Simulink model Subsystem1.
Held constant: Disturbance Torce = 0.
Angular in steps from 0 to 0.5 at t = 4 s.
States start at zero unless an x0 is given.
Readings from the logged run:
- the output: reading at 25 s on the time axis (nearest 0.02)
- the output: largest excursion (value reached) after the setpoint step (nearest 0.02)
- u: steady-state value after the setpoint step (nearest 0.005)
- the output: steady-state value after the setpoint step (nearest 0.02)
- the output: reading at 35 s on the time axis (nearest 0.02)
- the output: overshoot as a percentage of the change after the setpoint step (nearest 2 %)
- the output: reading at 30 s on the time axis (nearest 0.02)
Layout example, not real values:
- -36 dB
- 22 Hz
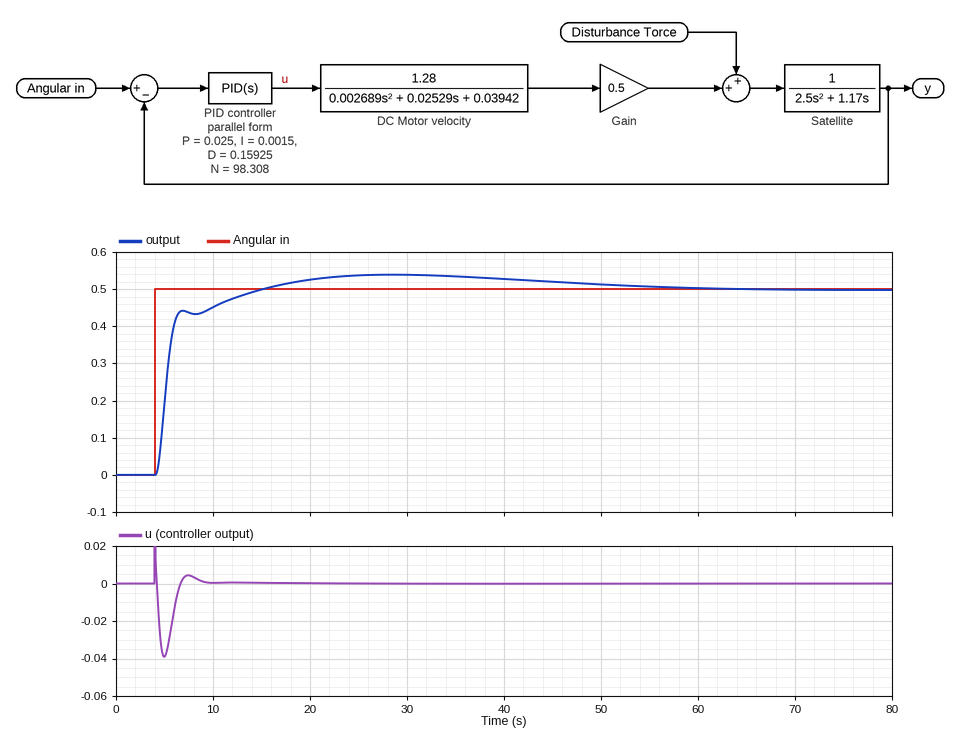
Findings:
- 0.54
- 0.54
- 0.000
- 0.50
- 0.54
- 8 %
- 0.54
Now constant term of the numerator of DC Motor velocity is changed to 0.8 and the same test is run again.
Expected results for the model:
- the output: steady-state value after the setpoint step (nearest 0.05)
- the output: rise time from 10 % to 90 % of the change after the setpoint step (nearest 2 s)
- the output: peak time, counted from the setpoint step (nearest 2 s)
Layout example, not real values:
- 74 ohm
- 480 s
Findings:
- 0.50
- 8 s
- 28 s
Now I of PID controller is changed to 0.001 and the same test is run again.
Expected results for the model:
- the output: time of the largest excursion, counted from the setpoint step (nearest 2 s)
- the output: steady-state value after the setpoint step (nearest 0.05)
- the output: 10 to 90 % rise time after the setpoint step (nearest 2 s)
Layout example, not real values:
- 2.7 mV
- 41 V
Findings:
- 28 s
- 0.50
- 6 s
